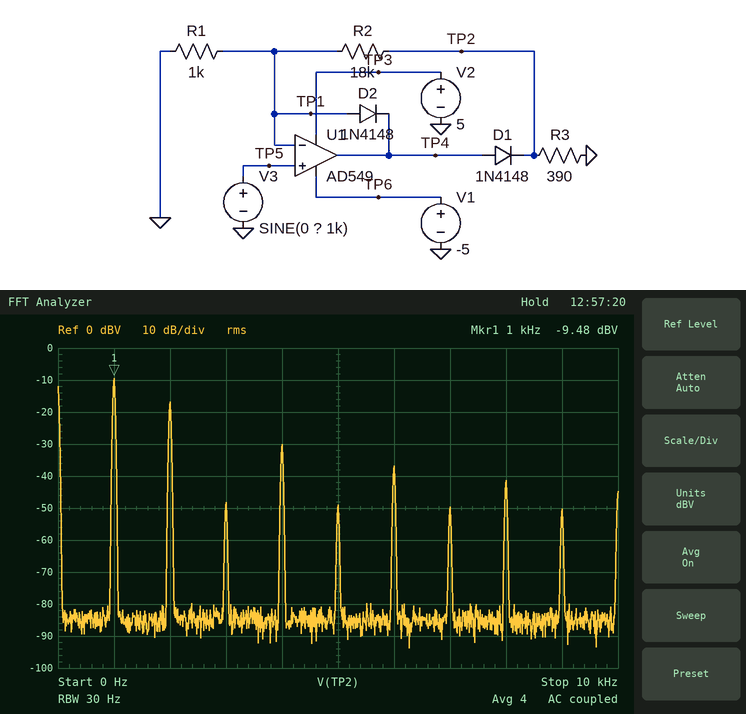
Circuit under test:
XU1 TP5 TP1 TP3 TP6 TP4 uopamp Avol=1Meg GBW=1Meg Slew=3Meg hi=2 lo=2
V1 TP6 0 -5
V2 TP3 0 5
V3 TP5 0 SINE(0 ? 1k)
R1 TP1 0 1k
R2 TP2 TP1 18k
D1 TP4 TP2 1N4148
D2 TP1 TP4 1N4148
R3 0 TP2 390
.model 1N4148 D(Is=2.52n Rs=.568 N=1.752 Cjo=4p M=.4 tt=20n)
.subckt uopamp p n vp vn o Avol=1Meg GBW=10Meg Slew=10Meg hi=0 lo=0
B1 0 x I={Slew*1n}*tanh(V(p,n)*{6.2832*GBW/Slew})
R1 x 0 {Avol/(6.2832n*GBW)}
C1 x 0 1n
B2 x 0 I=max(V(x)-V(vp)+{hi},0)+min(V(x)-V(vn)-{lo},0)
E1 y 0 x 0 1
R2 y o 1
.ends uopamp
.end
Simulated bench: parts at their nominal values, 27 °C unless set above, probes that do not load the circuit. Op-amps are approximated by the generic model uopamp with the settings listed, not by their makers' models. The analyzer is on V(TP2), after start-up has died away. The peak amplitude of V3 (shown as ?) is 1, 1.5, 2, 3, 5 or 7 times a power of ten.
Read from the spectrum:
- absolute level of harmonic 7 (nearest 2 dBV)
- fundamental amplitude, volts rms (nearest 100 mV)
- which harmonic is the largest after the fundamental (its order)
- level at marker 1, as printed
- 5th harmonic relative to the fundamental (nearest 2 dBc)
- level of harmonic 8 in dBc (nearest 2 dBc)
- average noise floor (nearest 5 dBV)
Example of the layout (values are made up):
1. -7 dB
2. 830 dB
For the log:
1. -50 dBV
2. 300 mV
3. 2
4. -9.48 dBV
5. -40 dBc
6. -32 dBc
7. -85 dBV
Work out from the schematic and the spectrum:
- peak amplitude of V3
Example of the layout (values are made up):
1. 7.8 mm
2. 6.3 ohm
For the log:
1. 50 mV
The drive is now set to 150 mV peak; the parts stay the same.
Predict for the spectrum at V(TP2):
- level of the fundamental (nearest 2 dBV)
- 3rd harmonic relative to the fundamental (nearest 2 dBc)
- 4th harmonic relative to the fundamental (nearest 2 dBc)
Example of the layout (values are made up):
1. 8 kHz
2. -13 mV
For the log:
1. 0 dBV
2. -22 dBc
3. -16 dBc
